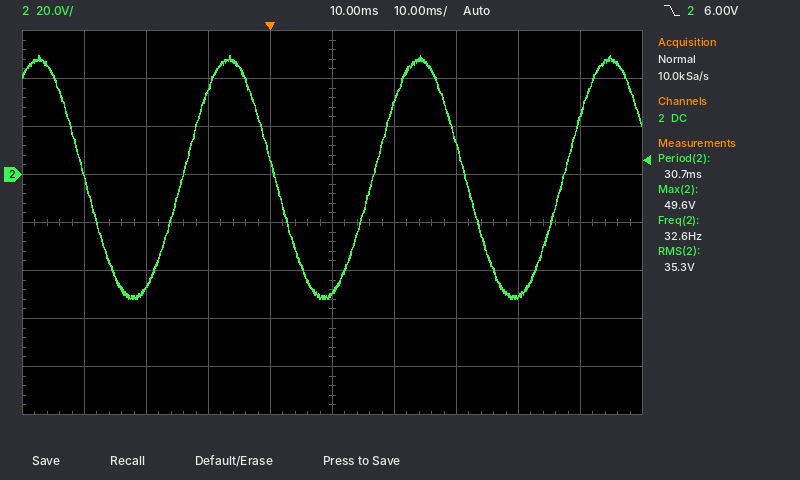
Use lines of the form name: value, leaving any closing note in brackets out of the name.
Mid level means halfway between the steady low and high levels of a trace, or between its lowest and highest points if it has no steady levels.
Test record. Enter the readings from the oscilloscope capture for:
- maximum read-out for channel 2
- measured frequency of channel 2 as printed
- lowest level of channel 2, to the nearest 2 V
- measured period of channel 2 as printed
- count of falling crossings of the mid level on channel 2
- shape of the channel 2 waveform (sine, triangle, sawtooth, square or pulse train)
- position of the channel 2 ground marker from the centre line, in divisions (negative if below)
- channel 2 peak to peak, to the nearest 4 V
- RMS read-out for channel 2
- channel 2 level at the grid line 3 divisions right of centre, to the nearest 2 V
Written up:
maximum read-out for channel 2: 49.6 V
measured frequency of channel 2 as printed: 32.6 Hz
lowest level of channel 2, to the nearest 2 V: -52 V
measured period of channel 2 as printed: 30.7 ms
count of falling crossings of the mid level on channel 2: 3
shape of the channel 2 waveform: sine
position of the channel 2 ground marker from the centre line, in divisions: +1.0 div
channel 2 peak to peak, to the nearest 4 V: 100 V
RMS read-out for channel 2: 35.3 V
channel 2 level at the grid line 3 divisions right of centre, to the nearest 2 V: -50 V
